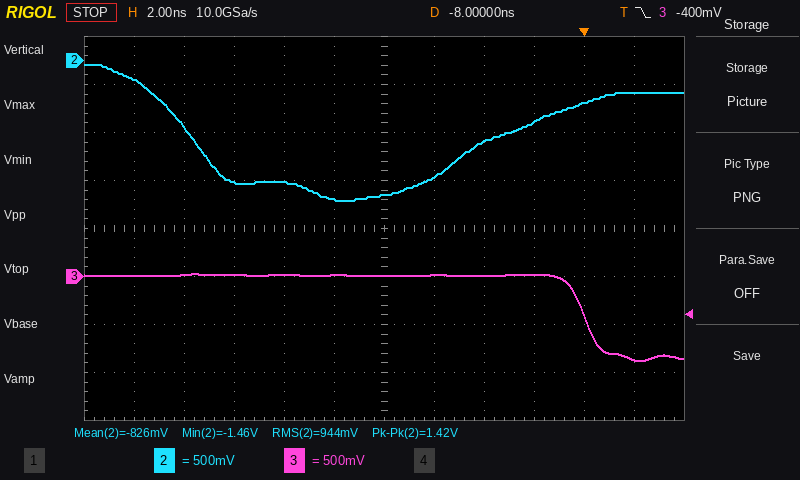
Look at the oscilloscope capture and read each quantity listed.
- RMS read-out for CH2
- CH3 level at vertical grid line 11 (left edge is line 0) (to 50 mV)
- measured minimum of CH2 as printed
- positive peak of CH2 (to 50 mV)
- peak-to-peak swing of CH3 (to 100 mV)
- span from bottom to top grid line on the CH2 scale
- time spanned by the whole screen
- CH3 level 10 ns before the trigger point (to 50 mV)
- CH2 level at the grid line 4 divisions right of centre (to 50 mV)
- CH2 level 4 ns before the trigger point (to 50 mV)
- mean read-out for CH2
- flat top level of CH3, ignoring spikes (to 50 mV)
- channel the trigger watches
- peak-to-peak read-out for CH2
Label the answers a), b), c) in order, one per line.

a) 944 mV
b) -850 mV
c) -1.46 V
d) -50 mV
e) 900 mV
f) 4 V
g) 24 ns
h) 0 mV
i) -450 mV
j) -850 mV
k) -826 mV
l) 0 mV
m) CH3
n) 1.42 V
